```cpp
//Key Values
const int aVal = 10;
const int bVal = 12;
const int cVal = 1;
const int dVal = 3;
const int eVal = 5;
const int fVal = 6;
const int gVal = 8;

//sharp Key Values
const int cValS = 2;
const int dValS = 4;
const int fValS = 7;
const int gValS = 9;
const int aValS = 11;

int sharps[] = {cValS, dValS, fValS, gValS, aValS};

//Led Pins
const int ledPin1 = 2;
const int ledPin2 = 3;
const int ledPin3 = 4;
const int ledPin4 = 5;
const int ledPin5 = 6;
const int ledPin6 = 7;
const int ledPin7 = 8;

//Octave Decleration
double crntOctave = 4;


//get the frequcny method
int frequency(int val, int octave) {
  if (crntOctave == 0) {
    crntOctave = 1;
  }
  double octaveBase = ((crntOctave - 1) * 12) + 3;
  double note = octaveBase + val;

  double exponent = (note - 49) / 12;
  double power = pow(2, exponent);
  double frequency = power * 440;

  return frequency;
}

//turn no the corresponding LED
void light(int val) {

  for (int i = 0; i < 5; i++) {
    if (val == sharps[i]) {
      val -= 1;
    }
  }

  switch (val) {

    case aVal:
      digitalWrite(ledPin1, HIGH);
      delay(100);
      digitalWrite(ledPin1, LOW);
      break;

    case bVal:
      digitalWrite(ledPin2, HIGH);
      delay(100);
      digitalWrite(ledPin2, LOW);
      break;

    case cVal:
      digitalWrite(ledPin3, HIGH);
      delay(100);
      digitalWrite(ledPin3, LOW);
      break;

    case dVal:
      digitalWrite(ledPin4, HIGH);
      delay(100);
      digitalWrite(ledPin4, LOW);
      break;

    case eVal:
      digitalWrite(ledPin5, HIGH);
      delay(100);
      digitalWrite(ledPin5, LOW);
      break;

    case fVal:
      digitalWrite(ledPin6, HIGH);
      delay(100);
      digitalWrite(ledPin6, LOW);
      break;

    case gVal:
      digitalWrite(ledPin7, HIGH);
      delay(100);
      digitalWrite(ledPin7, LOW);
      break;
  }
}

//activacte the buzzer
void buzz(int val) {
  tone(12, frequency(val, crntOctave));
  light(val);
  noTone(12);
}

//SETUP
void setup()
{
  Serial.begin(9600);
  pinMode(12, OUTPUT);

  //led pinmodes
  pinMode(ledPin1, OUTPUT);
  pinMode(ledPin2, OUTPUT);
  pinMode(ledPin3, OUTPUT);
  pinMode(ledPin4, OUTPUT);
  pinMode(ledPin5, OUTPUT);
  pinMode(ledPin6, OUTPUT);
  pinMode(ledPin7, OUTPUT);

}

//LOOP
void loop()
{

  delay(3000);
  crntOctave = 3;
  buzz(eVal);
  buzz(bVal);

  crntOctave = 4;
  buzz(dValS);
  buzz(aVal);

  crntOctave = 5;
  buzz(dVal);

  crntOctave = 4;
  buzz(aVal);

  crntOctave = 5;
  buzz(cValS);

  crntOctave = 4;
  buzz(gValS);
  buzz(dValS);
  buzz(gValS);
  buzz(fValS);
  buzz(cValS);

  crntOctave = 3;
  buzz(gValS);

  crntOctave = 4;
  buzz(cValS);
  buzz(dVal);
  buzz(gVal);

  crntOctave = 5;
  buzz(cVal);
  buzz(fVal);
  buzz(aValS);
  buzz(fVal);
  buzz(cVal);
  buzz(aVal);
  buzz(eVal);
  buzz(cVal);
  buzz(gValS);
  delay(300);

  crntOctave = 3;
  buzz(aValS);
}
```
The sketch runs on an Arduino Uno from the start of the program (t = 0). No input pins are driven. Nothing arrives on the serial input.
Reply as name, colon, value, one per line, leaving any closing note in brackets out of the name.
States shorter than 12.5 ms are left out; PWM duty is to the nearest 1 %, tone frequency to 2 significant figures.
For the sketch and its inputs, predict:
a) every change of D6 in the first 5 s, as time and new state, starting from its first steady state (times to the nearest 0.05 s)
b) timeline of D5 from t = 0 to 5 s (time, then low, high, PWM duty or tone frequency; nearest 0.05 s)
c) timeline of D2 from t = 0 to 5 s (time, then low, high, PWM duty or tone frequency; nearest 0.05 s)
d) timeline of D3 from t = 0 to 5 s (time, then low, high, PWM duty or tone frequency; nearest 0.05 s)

every change of D6 in the first 5 s, as time and new state, starting from its first steady state: 0 s low; 3 s high; 3.1 s low
timeline of D5 from t = 0 to 5 s: 0 s low; 3.2 s high; 3.3 s low; 3.4 s high; 3.5 s low; 3.8 s high; 3.9 s low; 4.4 s high; 4.5 s low
timeline of D2 from t = 0 to 5 s: 0 s low; 3.3 s high; 3.4 s low; 3.5 s high; 3.6 s low; 4.8 s high; 4.9 s low
timeline of D3 from t = 0 to 5 s: 0 s low; 3.1 s high; 3.2 s low
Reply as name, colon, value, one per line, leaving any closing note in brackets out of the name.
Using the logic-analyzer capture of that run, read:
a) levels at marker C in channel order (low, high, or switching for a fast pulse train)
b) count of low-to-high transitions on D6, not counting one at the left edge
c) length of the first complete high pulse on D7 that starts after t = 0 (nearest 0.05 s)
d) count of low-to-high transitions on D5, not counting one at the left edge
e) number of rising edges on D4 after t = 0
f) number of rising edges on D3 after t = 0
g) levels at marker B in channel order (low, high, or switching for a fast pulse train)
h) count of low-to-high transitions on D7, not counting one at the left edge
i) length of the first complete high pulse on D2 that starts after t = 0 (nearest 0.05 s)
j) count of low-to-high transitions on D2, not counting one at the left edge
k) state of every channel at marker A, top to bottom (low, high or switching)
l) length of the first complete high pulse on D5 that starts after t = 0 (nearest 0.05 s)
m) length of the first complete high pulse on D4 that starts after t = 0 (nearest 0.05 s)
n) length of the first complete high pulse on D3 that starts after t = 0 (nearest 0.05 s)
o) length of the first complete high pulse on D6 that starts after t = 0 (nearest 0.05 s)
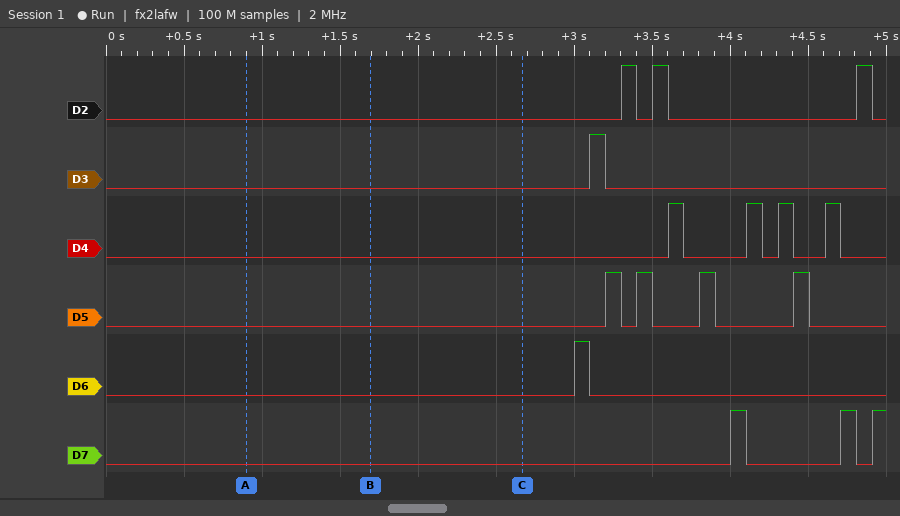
levels at marker C in channel order: D2 low, D3 low, D4 low, D5 low, D6 low, D7 low
count of low-to-high transitions on D6, not counting one at the left edge: 1
length of the first complete high pulse on D7 that starts after t = 0: 0.10 s
count of low-to-high transitions on D5, not counting one at the left edge: 4
number of rising edges on D4 after t = 0: 4
number of rising edges on D3 after t = 0: 1
levels at marker B in channel order: D2 low, D3 low, D4 low, D5 low, D6 low, D7 low
count of low-to-high transitions on D7, not counting one at the left edge: 3
length of the first complete high pulse on D2 that starts after t = 0: 0.10 s
count of low-to-high transitions on D2, not counting one at the left edge: 3
state of every channel at marker A, top to bottom: D2 low, D3 low, D4 low, D5 low, D6 low, D7 low
length of the first complete high pulse on D5 that starts after t = 0: 0.10 s
length of the first complete high pulse on D4 that starts after t = 0: 0.10 s
length of the first complete high pulse on D3 that starts after t = 0: 0.10 s
length of the first complete high pulse on D6 that starts after t = 0: 0.10 s
